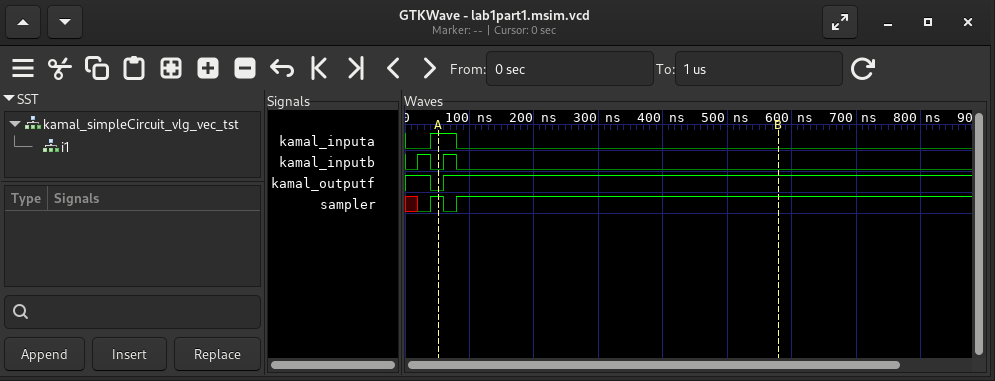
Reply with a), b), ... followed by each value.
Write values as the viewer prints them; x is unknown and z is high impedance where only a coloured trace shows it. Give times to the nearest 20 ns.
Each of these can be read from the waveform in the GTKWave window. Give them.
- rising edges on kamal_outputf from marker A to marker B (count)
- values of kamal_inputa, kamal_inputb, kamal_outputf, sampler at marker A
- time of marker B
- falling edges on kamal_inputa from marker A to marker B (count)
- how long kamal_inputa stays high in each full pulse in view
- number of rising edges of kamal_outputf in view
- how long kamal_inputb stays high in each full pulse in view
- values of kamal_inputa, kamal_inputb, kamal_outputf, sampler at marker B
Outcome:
a) 1
b) kamal_inputa=1, kamal_inputb=0, kamal_outputf=0, sampler=1
c) 580 ns
d) 1
e) 40 ns
f) 1
g) 20 ns, 20 ns
h) kamal_inputa=0, kamal_inputb=0, kamal_outputf=1, sampler=1
